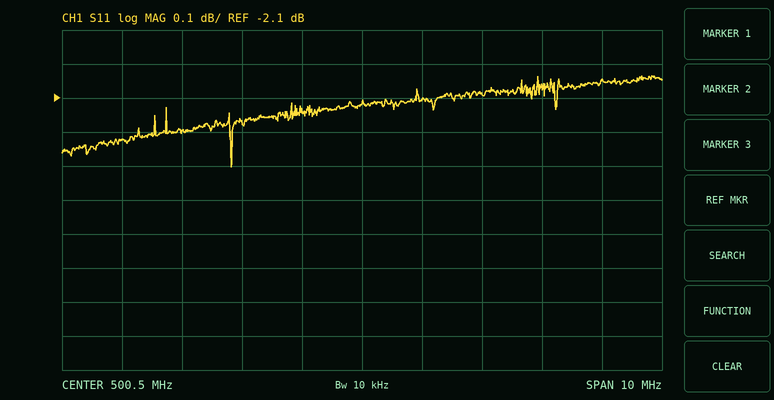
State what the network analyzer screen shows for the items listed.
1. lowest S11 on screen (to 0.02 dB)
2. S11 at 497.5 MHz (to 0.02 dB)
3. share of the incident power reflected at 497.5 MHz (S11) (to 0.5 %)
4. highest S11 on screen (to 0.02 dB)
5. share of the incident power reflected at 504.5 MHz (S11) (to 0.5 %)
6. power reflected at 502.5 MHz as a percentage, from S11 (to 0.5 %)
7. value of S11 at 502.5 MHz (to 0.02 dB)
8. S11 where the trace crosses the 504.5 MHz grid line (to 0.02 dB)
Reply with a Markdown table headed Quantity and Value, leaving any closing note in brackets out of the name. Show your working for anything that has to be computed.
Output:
| Quantity | Value |
|---|---|
| lowest S11 on screen | -2.30 dB |
| S11 at 497.5 MHz | -2.20 dB |
| share of the incident power reflected at 497.5 MHz (S11) | 10^(-2.2/10) ≈ 60.3 %, so 60.5 % to the nearest 0.5 % |
| highest S11 on screen | -2.04 dB |
| share of the incident power reflected at 504.5 MHz (S11) | 10^(-2.04/10) ≈ 62.5 % |
| power reflected at 502.5 MHz as a percentage, from S11 | 10^(-2.08/10) ≈ 61.9 %, so 62.0 % to the nearest 0.5 % |
| value of S11 at 502.5 MHz | -2.08 dB |
| S11 where the trace crosses the 504.5 MHz grid line | -2.04 dB |
